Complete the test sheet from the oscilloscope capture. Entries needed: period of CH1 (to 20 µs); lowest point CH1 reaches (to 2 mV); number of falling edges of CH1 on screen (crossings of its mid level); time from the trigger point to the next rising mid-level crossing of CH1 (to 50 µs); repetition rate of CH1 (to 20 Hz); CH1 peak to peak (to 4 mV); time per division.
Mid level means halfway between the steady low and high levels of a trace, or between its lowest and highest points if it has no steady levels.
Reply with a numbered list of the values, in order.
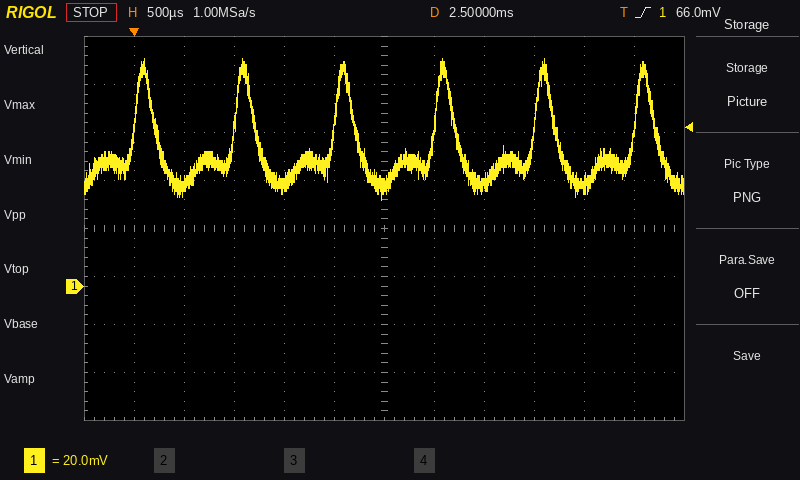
1. 1.00 ms
2. 36 mV
3. 6
4. 1.00 ms
5. 1.00 kHz
6. 60 mV
7. 500 µs
